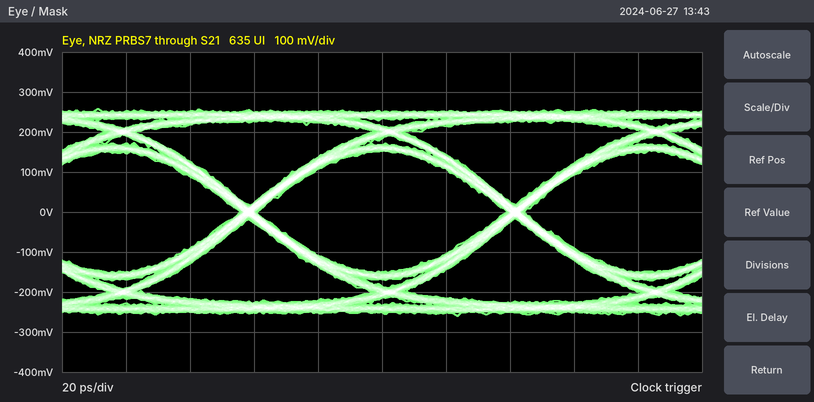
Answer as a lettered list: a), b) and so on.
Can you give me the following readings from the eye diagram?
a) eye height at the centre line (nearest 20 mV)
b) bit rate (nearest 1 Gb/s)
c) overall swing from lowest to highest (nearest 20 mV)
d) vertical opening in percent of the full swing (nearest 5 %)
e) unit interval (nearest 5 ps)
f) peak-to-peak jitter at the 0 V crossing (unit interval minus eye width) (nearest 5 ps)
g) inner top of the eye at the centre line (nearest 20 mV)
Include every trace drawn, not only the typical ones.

a) 300 mV
b) 12 Gb/s
c) 520 mV
d) 60 %
e) 85 ps
f) 5 ps
g) 160 mV
